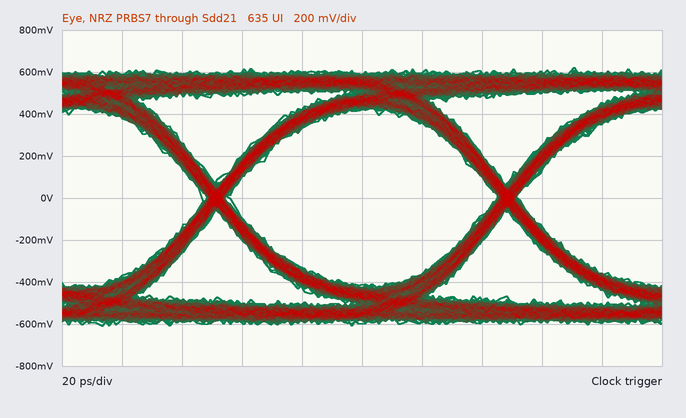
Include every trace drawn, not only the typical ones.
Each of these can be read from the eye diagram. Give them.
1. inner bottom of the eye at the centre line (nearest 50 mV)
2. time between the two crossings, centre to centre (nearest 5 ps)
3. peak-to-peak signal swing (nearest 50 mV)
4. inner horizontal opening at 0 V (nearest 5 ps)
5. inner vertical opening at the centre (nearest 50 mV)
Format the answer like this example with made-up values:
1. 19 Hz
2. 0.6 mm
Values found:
1. -400 mV
2. 95 ps
3. 1.25 V
4. 90 ps
5. 850 mV
